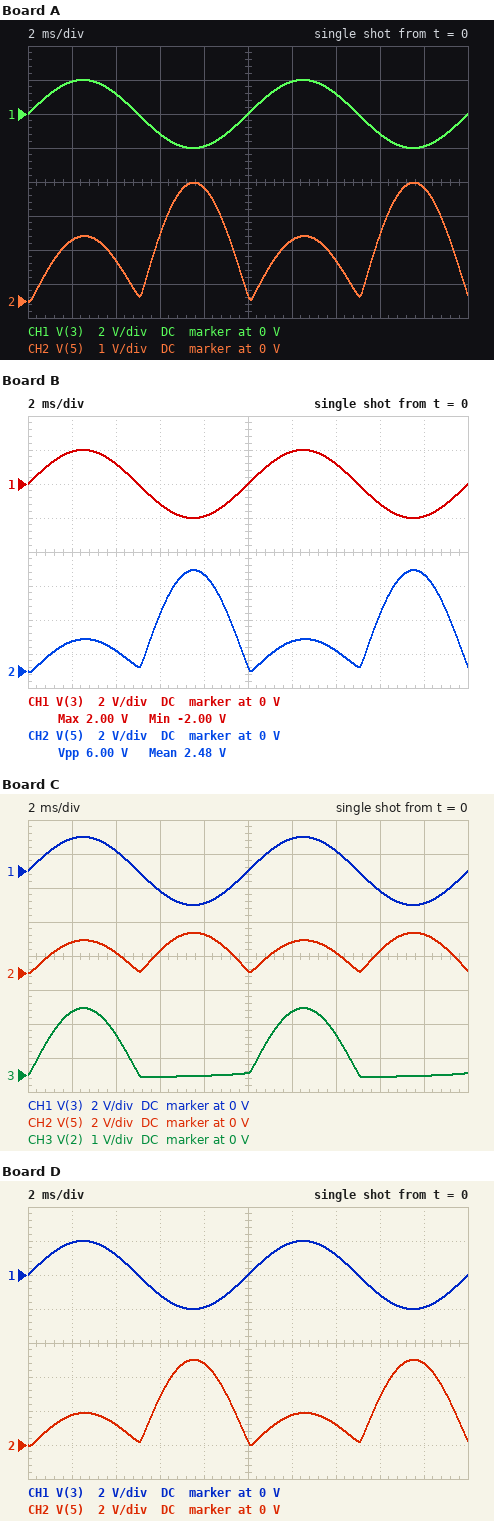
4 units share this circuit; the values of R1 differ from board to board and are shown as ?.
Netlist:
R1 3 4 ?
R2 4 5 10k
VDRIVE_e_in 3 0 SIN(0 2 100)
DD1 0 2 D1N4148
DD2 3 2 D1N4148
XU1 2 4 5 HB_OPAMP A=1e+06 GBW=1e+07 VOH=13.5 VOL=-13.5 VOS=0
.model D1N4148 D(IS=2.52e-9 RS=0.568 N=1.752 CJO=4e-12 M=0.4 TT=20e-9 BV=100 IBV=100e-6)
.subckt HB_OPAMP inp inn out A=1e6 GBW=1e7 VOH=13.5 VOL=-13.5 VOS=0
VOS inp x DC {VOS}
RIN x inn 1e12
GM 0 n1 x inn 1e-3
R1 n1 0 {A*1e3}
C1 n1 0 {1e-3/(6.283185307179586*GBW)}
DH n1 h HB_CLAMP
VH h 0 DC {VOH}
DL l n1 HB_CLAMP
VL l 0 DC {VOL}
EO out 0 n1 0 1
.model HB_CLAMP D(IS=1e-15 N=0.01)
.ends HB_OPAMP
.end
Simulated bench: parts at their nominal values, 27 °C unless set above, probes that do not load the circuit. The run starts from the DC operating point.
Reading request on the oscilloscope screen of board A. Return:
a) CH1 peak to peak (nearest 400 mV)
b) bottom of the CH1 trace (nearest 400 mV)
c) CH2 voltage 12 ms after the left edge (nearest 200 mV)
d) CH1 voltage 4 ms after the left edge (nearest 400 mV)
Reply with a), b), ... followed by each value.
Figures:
a) 4.0 V
b) -2.0 V
c) 1.8 V
d) 1.2 V
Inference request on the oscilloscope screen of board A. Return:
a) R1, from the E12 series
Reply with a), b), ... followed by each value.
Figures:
a) 5.6 kΩ
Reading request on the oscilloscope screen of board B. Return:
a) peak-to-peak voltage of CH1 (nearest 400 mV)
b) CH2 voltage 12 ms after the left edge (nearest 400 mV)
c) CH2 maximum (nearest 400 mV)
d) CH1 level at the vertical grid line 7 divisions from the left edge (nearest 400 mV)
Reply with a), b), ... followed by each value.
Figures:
a) 4.0 V
b) 1.6 V
c) 6.0 V
d) 1.2 V
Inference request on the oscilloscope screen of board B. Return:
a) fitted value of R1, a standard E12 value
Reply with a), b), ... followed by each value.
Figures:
a) 3.3 kΩ
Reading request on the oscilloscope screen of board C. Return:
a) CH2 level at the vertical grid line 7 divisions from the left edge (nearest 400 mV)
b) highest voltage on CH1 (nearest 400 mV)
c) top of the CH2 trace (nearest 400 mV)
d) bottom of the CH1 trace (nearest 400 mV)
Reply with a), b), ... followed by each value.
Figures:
a) 1.2 V
b) 2.0 V
c) 2.4 V
d) -2.0 V
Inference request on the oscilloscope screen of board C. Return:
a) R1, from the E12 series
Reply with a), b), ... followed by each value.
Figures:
a) 8.2 kΩ
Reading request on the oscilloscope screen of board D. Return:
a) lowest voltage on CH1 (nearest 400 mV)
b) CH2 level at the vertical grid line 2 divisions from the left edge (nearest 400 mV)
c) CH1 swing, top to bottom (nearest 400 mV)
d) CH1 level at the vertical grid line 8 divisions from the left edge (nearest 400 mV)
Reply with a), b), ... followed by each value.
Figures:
a) -2.0 V
b) 1.2 V
c) 4.0 V
d) -1.2 V
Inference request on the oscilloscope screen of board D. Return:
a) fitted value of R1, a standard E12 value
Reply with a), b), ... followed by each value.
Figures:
a) 3.9 kΩ
